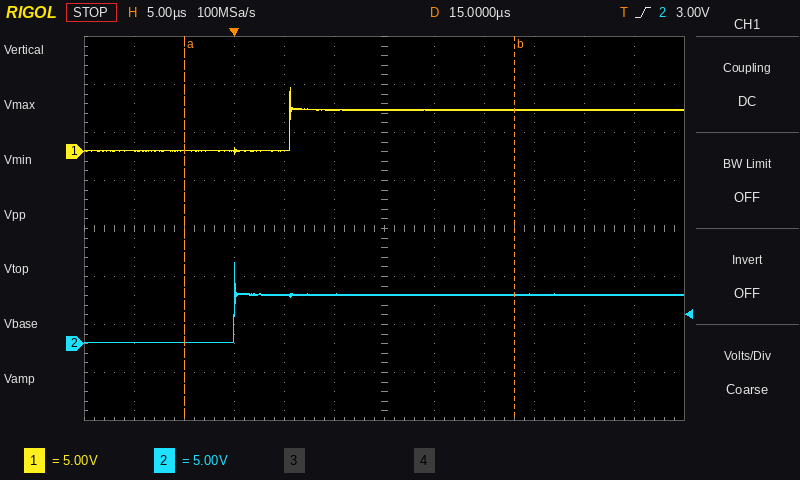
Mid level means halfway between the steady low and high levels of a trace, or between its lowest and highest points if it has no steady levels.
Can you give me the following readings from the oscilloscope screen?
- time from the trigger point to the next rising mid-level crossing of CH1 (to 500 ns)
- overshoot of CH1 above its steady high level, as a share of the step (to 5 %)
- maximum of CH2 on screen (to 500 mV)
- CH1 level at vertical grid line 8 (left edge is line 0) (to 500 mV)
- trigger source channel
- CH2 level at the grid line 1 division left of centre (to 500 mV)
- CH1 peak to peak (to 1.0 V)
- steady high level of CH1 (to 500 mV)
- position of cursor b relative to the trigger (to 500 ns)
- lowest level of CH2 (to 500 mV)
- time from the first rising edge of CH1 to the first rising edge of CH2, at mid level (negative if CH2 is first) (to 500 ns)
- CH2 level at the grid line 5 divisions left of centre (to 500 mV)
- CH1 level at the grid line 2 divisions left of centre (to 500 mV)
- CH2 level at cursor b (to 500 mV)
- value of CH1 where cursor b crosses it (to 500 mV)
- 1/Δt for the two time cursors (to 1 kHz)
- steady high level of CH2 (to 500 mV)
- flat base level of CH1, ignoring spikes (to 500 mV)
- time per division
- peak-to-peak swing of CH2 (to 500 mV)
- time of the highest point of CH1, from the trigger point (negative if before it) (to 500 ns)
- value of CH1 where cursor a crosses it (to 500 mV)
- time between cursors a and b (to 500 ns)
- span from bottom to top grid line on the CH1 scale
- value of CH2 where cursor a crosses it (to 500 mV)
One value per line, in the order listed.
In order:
5.5 µs
55 %
8.5 V
4.5 V
CH2
5.0 V
7.0 V
4.5 V
+28.0 µs
0.0 V
-5.5 µs
0.0 V
0.0 V
5.0 V
4.5 V
30 kHz
5.0 V
0.0 V
5 µs
8.5 V
+5.5 µs
0.0 V
33.0 µs
40 V
0.0 V
